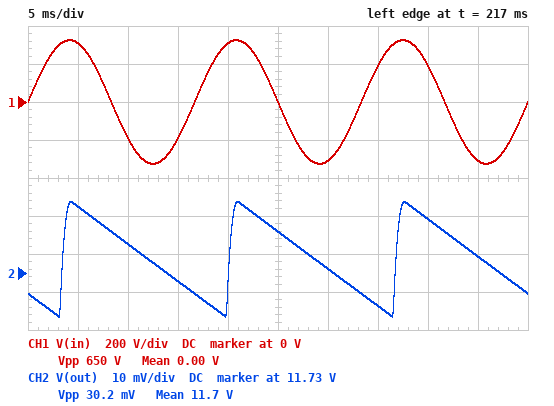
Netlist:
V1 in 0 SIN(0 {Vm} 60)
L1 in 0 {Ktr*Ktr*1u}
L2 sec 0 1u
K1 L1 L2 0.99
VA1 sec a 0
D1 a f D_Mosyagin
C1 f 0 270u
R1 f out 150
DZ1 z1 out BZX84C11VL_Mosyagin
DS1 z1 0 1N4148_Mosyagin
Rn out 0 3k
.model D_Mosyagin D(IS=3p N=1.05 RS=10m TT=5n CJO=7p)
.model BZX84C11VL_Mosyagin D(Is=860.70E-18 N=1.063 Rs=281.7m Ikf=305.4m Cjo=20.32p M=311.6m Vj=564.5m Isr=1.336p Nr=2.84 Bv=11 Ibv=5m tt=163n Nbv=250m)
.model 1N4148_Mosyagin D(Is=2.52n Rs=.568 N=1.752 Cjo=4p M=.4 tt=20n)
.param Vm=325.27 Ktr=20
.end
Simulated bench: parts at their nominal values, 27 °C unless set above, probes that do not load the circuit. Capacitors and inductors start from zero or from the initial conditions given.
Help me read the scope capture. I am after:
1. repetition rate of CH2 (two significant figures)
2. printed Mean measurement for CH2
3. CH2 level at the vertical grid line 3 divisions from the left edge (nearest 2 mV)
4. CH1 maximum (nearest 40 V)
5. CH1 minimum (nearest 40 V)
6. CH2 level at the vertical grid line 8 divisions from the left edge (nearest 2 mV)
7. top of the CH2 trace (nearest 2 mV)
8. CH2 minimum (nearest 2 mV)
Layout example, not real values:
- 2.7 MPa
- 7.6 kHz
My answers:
- 60 Hz
- 11.7 V
- 11.728 V
- 320 V
- -320 V
- 11.744 V
- 11.748 V
- 11.718 V
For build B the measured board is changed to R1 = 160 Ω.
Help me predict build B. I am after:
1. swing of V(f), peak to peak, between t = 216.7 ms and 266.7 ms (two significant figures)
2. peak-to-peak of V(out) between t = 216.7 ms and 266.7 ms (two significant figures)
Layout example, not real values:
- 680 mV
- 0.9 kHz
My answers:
- 1.1 V
- 28 mV
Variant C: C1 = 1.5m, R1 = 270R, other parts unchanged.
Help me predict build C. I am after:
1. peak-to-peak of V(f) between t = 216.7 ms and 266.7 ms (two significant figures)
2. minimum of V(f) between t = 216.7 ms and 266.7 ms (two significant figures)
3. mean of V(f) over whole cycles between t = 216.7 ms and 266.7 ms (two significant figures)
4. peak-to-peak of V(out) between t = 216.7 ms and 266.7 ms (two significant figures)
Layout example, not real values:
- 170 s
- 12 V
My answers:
- 140 mV
- 15 V
- 15 V
- 3.2 mV
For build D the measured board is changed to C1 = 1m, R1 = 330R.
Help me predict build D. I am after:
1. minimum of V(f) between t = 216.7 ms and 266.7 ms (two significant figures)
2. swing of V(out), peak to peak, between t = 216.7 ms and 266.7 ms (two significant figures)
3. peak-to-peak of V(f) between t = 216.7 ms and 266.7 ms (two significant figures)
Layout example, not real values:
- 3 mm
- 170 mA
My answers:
- 15 V
- 4.2 mV
- 180 mV
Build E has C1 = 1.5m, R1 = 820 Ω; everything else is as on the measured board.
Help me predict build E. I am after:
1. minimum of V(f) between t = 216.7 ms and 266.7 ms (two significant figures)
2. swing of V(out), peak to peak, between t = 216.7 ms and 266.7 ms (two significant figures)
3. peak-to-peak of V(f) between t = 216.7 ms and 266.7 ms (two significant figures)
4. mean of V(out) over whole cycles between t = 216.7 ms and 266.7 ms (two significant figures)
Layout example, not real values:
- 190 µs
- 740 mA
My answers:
- 15 V
- 3.5 mV
- 50 mV
- 12 V
